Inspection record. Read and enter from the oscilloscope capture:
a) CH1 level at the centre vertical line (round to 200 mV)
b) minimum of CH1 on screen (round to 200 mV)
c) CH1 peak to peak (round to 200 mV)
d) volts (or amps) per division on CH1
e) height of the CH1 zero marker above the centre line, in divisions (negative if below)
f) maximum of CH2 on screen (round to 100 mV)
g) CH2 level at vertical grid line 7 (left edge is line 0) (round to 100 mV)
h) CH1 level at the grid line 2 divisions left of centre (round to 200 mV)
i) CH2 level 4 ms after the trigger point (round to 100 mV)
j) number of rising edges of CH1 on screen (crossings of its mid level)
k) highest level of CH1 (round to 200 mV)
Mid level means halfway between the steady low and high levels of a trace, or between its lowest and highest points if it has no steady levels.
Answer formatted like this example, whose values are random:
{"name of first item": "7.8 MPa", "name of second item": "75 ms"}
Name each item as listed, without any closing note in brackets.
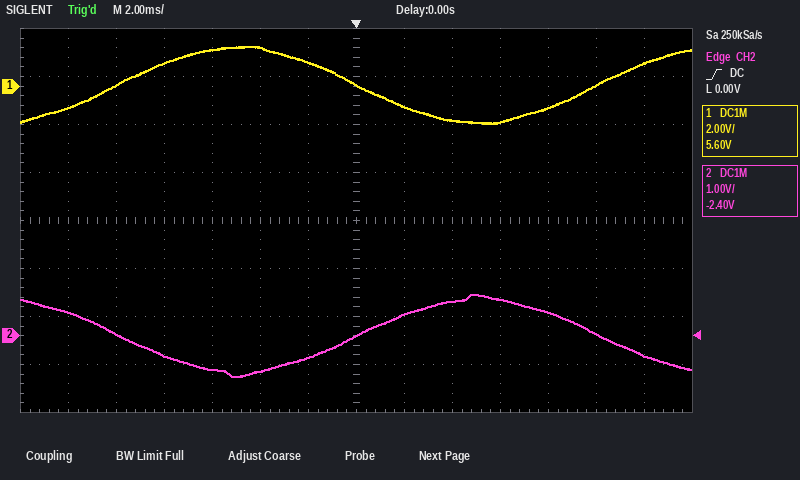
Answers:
{"CH1 level at the centre vertical line": "0.0 V", "minimum of CH1 on screen": "-1.6 V", "CH1 peak to peak": "3.2 V", "volts (or amps) per division on CH1": "2 V", "height of the CH1 zero marker above the centre line, in divisions": "+2.8 div", "maximum of CH2 on screen": "900 mV", "CH2 level at vertical grid line 7 (left edge is line 0)": "0.0 V", "CH1 level at the grid line 2 divisions left of centre": "1.6 V", "CH2 level 4 ms after the trigger point": "700 mV", "number of rising edges of CH1 on screen": "2", "highest level of CH1": "1.6 V"}
